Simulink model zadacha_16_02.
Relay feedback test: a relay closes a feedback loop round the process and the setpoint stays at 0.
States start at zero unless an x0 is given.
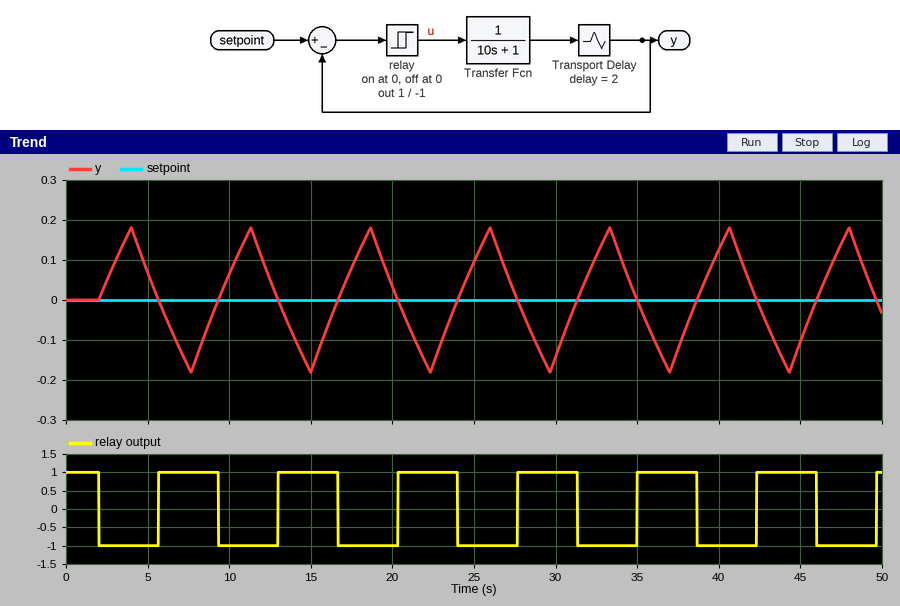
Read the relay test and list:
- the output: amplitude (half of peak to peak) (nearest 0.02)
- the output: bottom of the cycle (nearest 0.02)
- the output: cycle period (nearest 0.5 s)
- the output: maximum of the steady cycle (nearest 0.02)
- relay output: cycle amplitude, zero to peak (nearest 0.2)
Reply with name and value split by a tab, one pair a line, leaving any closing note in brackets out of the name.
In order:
the output: amplitude (half of peak to peak)	0.18
the output: bottom of the cycle	-0.18
the output: cycle period	7.5 s
the output: maximum of the steady cycle	0.18
relay output: cycle amplitude, zero to peak	1.0
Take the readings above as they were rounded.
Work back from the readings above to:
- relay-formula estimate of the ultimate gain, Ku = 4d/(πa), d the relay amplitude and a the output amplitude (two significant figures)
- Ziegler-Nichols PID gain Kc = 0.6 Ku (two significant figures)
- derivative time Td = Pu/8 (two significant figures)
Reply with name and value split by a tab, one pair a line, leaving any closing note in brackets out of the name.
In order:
relay-formula estimate of the ultimate gain, Ku = 4d/(πa), d the relay amplitude and a the output amplitude	7.1
Ziegler-Nichols PID gain Kc = 0.6 Ku	4.3
derivative time Td = Pu/8	0.94 s
